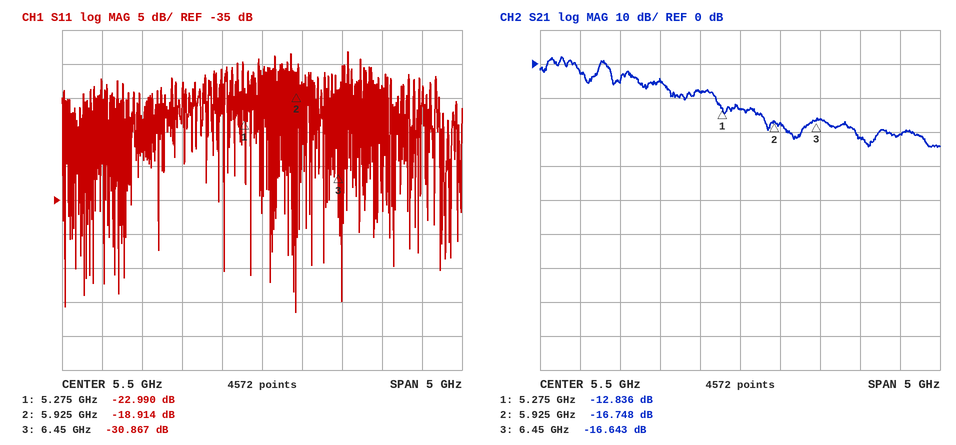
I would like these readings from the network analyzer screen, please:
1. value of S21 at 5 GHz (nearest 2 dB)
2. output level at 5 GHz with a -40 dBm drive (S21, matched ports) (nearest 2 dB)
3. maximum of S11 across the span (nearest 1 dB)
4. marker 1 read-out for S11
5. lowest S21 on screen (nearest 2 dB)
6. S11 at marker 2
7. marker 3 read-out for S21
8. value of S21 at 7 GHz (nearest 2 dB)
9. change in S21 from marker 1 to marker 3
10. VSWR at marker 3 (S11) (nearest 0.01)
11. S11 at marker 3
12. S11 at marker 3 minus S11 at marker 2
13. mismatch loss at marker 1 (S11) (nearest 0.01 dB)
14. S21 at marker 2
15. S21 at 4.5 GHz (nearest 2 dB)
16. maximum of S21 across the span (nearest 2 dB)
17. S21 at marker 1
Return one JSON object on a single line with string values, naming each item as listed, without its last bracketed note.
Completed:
{"value of S21 at 5 GHz": "-8 dB", "output level at 5 GHz with a -40 dBm drive (S21, matched ports)": "-48 dBm", "maximum of S11 across the span": "-13 dB", "marker 1 read-out for S11": "-22.990 dB", "lowest S21 on screen": "-24 dB", "S11 at marker 2": "-18.914 dB", "marker 3 read-out for S21": "-16.643 dB", "value of S21 at 7 GHz": "-22 dB", "change in S21 from marker 1 to marker 3": "-3.807 dB", "VSWR at marker 3 (S11)": "1.06", "S11 at marker 3": "-30.867 dB", "S11 at marker 3 minus S11 at marker 2": "-11.953 dB", "mismatch loss at marker 1 (S11)": "0.02 dB", "S21 at marker 2": "-16.748 dB", "S21 at 4.5 GHz": "-4 dB", "maximum of S21 across the span": "2 dB", "S21 at marker 1": "-12.836 dB"}
